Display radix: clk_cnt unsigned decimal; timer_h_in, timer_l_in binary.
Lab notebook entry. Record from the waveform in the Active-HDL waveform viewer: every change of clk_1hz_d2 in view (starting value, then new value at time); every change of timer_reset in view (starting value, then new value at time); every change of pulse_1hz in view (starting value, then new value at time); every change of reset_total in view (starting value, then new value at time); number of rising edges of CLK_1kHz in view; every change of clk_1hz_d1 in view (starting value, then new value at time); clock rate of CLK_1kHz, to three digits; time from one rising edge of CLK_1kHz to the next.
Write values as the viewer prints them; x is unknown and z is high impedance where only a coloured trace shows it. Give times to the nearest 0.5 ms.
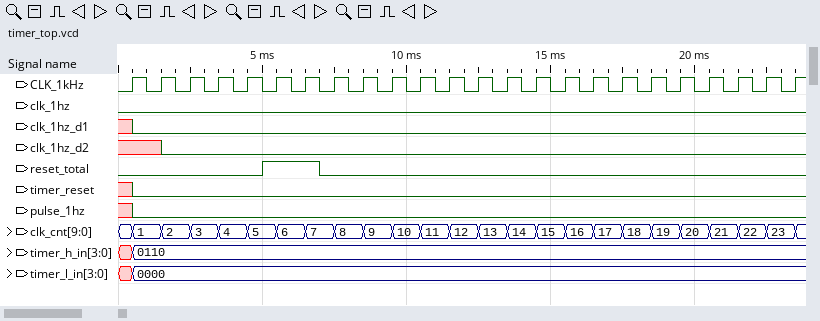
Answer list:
x, 0 at 1.5 ms
x, 0 at 0.5 ms
x, 0 at 0.5 ms
0, 1 at 5 ms, 0 at 7 ms
24
x, 0 at 0.5 ms
1.00 kHz
1 ms
